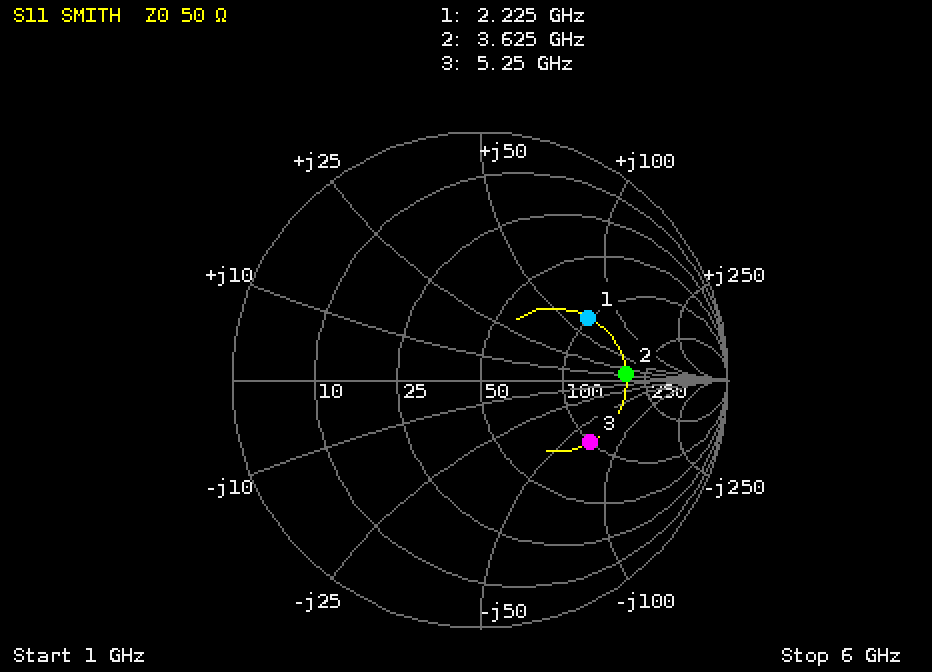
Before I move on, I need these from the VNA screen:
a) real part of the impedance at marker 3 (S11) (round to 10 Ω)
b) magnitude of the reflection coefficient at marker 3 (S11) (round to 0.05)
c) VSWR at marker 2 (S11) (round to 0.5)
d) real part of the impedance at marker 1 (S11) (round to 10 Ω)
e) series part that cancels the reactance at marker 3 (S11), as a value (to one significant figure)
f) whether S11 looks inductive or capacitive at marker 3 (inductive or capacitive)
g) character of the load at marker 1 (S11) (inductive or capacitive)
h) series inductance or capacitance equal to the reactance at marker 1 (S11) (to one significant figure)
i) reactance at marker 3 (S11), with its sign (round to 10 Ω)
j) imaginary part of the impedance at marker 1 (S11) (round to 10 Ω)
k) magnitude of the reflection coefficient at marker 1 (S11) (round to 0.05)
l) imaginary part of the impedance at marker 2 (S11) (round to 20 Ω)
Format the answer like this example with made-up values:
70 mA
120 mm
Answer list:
100 Ω
0.50
4.0
100 Ω
2 nH
capacitive
inductive
5 nH
-70 Ω
+70 Ω
0.50
+20 Ω
